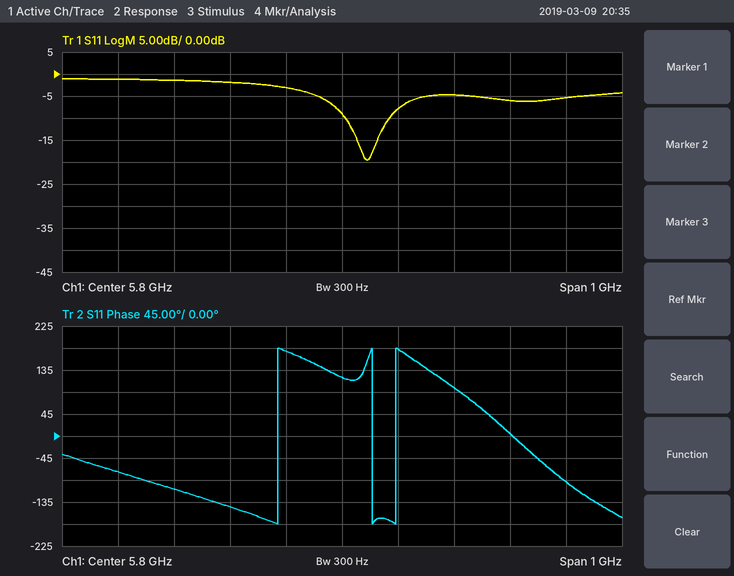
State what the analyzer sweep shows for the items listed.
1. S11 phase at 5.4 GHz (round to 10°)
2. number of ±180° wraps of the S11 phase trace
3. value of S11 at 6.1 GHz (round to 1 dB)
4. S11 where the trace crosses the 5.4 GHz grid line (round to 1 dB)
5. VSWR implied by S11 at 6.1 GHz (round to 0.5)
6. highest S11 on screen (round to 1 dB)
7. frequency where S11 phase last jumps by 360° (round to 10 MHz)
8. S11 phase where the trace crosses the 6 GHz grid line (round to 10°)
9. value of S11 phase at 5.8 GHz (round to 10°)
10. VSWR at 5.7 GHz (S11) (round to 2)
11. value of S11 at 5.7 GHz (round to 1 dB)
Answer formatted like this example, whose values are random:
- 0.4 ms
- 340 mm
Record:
- -70°
- 3
- -6 dB
- -1 dB
- 3.0
- -1 dB
- 5.90 GHz
- 100°
- 120°
- 6
- -3 dB
